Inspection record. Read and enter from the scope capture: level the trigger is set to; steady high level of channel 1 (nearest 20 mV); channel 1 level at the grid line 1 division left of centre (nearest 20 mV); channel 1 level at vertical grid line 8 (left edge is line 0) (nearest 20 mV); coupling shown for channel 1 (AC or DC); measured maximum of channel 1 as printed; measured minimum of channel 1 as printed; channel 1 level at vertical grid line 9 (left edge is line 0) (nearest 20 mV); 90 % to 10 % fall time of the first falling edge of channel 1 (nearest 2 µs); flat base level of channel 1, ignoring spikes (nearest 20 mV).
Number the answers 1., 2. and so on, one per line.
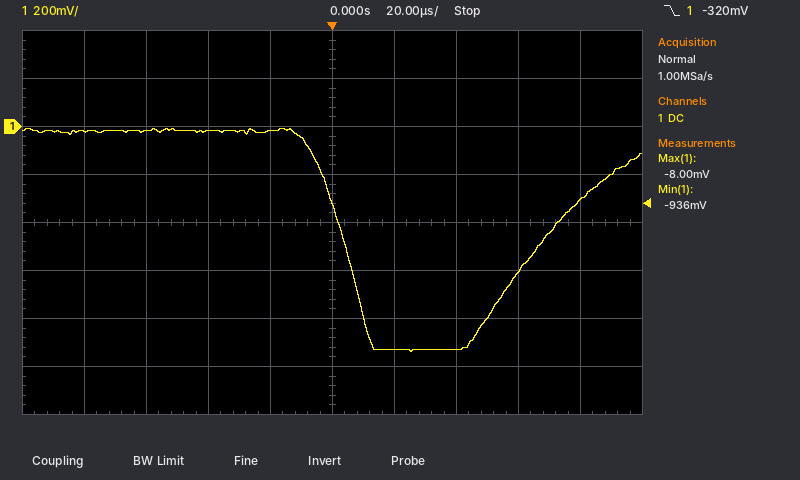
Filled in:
1. -320 mV
2. -20 mV
3. -20 mV
4. -600 mV
5. DC
6. -8.00 mV
7. -936 mV
8. -300 mV
9. 18 µs
10. -920 mV
